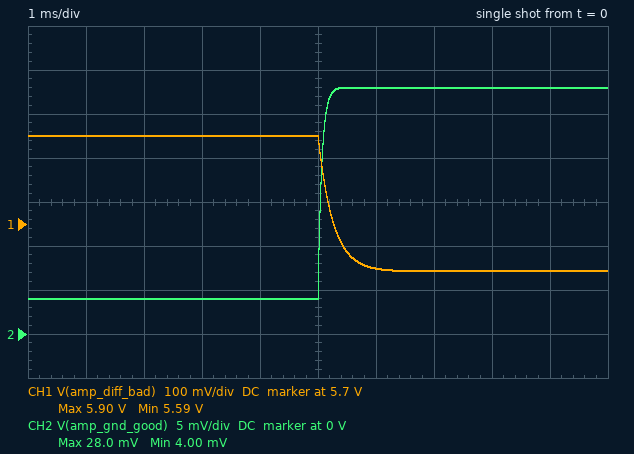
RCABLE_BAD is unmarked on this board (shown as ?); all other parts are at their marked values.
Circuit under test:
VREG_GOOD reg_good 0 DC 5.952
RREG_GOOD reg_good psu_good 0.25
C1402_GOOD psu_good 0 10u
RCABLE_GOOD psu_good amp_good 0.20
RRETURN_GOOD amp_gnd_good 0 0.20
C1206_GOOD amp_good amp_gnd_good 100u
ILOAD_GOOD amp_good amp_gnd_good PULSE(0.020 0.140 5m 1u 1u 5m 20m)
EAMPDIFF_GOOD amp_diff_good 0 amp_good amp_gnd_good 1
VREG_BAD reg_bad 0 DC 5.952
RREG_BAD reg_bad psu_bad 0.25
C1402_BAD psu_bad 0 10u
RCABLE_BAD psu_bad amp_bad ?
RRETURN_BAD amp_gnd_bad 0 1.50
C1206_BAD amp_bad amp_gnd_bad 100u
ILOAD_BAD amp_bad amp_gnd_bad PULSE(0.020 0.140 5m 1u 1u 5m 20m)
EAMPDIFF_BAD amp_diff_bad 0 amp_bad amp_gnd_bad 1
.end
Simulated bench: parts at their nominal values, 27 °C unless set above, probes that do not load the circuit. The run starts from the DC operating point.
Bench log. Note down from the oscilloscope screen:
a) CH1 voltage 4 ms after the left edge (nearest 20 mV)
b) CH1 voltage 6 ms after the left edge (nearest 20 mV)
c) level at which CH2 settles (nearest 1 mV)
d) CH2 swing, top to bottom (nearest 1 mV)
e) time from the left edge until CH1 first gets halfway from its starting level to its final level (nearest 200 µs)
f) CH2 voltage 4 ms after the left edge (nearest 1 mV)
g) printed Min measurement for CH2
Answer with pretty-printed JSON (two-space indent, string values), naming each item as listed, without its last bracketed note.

{
  "CH1 voltage 4 ms after the left edge": "5.90 V",
  "CH1 voltage 6 ms after the left edge": "5.60 V",
  "level at which CH2 settles": "28 mV",
  "CH2 swing, top to bottom": "24 mV",
  "time from the left edge until CH1 first gets halfway from its starting level to its final level": "5.2 ms",
  "CH2 voltage 4 ms after the left edge": "4 mV",
  "printed Min measurement for CH2": "4.00 mV"
}
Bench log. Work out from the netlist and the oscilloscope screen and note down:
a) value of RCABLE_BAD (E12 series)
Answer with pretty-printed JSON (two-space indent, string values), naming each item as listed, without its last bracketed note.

{
  "value of RCABLE_BAD": "0.82 Ω"
}
